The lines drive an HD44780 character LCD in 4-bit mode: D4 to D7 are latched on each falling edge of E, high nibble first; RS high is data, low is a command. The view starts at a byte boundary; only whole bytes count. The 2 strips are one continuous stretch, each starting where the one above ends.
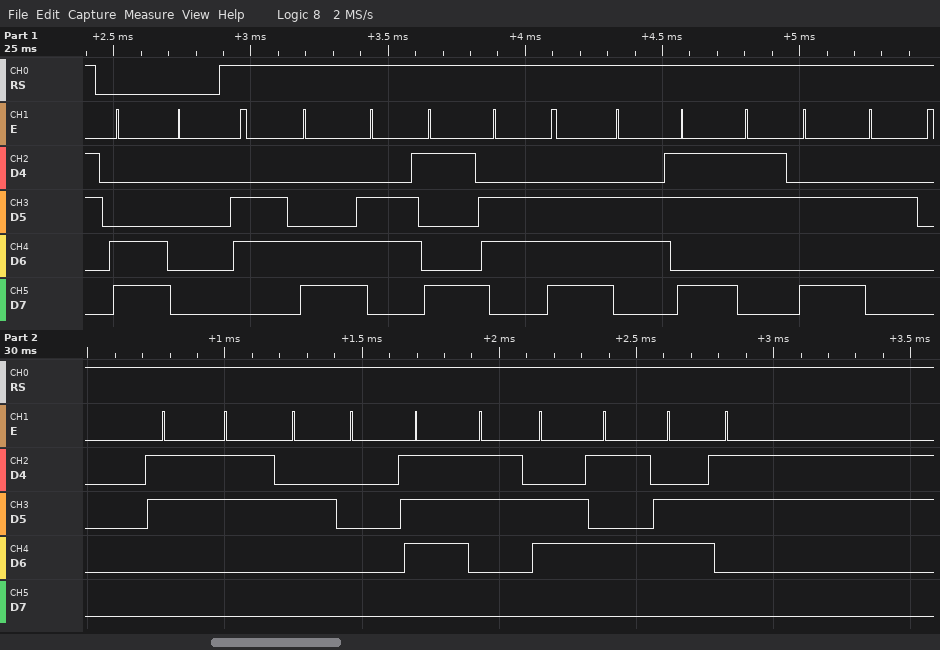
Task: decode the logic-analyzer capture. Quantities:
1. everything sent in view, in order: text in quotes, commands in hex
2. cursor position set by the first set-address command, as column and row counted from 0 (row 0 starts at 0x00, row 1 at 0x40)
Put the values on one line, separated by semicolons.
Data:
0xC0 "link: 3 sec"; column 0, row 1
